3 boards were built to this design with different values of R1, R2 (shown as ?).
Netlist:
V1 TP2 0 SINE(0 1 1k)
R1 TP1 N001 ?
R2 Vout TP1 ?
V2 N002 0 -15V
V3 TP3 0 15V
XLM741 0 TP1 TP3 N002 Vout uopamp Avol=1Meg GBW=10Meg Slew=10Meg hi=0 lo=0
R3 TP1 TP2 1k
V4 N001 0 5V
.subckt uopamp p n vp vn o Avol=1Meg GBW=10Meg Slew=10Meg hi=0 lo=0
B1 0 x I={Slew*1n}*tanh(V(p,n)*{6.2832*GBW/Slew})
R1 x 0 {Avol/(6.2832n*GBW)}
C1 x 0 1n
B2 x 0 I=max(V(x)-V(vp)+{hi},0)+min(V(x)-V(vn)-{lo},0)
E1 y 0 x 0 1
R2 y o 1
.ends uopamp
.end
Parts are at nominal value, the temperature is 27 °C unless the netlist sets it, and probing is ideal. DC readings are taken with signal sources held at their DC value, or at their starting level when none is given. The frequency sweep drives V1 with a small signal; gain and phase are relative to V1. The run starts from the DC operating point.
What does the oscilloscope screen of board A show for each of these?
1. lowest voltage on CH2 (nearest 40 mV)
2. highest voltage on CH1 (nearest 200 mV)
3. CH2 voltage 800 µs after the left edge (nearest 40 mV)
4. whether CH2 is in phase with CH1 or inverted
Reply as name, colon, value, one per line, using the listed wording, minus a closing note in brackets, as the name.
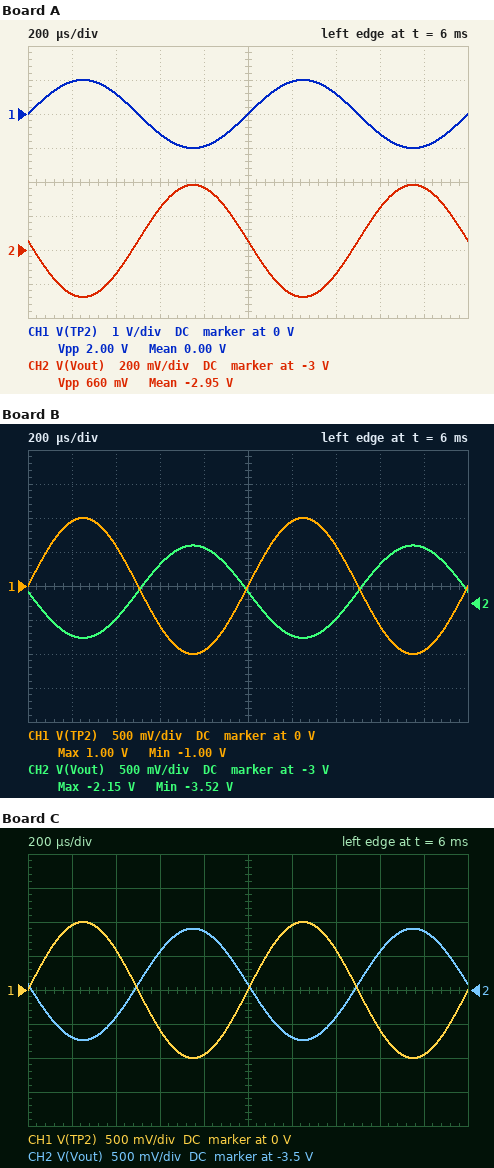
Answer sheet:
lowest voltage on CH2: -3.28 V
highest voltage on CH1: 1.0 V
CH2 voltage 800 µs after the left edge: -2.64 V
whether CH2 is in phase with CH1 or inverted: inverted
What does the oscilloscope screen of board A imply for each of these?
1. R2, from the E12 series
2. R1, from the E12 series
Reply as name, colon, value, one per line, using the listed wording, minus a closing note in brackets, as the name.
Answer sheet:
R2, from the E12 series: 330 Ω
R1, from the E12 series: 560 Ω
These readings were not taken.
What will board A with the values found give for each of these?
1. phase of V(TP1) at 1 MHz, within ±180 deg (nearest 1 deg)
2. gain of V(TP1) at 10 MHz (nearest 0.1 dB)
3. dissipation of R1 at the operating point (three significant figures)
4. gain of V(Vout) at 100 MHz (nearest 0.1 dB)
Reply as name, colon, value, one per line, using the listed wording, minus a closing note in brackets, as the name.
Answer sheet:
phase of V(TP1) at 1 MHz, within ±180 deg: 79 deg
gain of V(TP1) at 10 MHz: -16.3 dB
dissipation of R1 at the operating point: 44.6 mW
gain of V(Vout) at 100 MHz: -35.3 dB
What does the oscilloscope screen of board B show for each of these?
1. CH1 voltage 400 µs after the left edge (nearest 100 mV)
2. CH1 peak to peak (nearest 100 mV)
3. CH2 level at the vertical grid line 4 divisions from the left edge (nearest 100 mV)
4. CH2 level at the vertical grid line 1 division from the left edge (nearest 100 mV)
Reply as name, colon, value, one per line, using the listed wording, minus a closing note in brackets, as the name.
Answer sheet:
CH1 voltage 400 µs after the left edge: 600 mV
CH1 peak to peak: 2.0 V
CH2 level at the vertical grid line 4 divisions from the left edge: -2.2 V
CH2 level at the vertical grid line 1 division from the left edge: -3.5 V
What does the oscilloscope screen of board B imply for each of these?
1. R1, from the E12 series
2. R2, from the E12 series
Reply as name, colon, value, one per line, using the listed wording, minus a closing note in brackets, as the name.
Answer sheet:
R1, from the E12 series: 1.2 kΩ
R2, from the E12 series: 680 Ω
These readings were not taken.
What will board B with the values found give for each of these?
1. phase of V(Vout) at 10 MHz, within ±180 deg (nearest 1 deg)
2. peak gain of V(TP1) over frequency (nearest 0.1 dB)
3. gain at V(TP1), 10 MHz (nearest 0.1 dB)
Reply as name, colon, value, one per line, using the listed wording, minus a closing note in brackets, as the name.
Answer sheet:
phase of V(Vout) at 10 MHz, within ±180 deg: 114 deg
peak gain of V(TP1) over frequency: -10.4 dB
gain at V(TP1), 10 MHz: -11.2 dB
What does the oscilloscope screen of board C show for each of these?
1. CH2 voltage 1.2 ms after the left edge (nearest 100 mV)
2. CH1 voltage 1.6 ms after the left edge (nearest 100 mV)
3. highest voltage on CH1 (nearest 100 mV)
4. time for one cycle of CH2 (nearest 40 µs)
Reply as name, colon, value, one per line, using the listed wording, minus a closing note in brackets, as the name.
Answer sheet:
CH2 voltage 1.2 ms after the left edge: -4.2 V
CH1 voltage 1.6 ms after the left edge: -600 mV
highest voltage on CH1: 1.0 V
time for one cycle of CH2: 1.00 ms
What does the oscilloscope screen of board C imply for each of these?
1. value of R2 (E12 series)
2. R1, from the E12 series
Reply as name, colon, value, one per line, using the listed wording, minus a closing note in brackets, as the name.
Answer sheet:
value of R2: 820 Ω
R1, from the E12 series: 1.2 kΩ
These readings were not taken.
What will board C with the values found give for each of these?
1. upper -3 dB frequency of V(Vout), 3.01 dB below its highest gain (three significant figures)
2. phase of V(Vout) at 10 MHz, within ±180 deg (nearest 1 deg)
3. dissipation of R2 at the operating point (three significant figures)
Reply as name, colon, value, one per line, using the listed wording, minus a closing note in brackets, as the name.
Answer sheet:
upper -3 dB frequency of V(Vout), 3.01 dB below its highest gain: 3.99 MHz
phase of V(Vout) at 10 MHz, within ±180 deg: 112 deg
dissipation of R2 at the operating point: 14.2 mW
